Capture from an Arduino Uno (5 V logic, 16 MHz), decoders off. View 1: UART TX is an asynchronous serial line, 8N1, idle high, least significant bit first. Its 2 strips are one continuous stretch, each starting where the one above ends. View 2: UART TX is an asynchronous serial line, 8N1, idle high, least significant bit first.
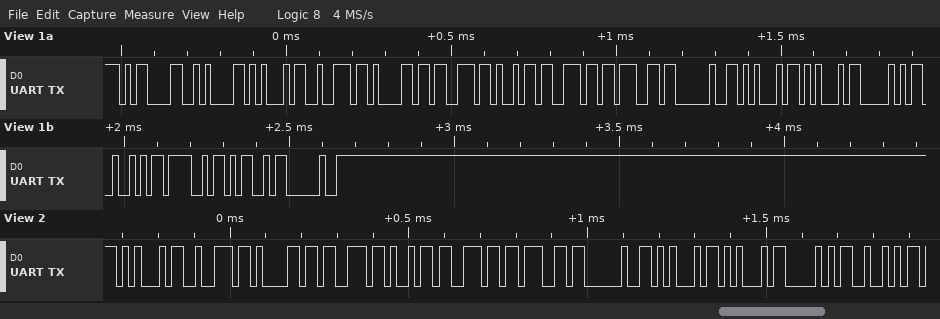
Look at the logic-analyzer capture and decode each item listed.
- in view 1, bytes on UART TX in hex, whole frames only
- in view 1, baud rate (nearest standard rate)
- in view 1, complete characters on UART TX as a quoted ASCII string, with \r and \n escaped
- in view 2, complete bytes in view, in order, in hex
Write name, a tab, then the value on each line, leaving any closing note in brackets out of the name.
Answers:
in view 1, bytes on UART TX in hex, whole frames only	0D 0A 45 72 61 73 69 6E 67 20 45 45 50 52 4F 4D 20
in view 1, baud rate	57600 baud
in view 1, complete characters on UART TX as a quoted ASCII string, with \r and \n escaped	"\r\nErasing EEPROM "
in view 2, complete bytes in view, in order, in hex	0x45 0x72 0x61 0x73 0x69 0x6E 0x67 0x20 0x45 0x45 0x50 0x52
